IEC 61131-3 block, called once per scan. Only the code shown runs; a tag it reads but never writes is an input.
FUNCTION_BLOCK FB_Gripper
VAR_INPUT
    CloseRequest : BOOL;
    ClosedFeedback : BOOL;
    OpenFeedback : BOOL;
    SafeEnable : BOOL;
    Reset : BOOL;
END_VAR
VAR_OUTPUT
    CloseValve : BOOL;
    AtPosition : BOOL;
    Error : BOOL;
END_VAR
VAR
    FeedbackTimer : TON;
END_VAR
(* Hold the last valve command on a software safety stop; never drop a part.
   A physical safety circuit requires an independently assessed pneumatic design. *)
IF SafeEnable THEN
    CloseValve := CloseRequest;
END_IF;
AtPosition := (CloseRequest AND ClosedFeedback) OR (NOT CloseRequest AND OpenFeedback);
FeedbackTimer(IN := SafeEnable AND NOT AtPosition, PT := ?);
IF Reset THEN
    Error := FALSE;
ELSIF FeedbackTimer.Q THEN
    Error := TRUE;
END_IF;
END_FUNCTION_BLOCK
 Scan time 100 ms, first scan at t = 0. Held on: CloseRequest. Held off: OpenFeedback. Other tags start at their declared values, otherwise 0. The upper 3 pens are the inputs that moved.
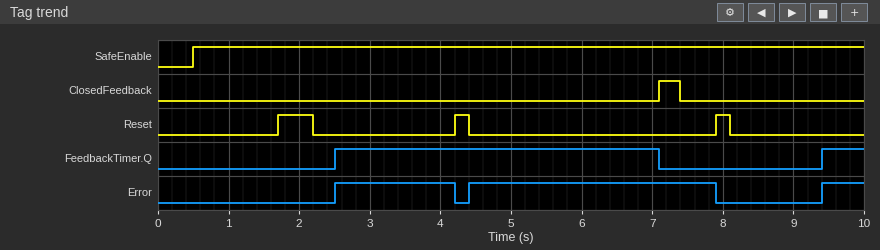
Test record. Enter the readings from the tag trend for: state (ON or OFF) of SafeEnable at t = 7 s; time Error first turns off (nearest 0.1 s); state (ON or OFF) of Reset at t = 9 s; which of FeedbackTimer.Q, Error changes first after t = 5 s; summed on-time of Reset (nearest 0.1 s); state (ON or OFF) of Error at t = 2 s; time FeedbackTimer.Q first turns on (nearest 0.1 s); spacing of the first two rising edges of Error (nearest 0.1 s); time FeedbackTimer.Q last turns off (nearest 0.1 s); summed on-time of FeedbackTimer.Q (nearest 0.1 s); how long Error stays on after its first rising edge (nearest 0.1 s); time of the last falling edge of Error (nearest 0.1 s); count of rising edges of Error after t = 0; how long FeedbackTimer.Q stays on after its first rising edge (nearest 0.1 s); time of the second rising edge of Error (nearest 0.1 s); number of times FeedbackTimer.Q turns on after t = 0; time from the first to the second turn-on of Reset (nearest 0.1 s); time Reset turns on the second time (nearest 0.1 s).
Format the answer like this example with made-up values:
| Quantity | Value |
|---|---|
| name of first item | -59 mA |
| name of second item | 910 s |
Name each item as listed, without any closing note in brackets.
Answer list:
| Quantity | Value |
|---|---|
| state (ON or OFF) of SafeEnable at t = 7 s | ON |
| time Error first turns off | 4.2 s |
| state (ON or OFF) of Reset at t = 9 s | OFF |
| which of FeedbackTimer.Q, Error changes first after t = 5 s | FeedbackTimer.Q |
| summed on-time of Reset | 0.9 s |
| state (ON or OFF) of Error at t = 2 s | OFF |
| time FeedbackTimer.Q first turns on | 2.5 s |
| spacing of the first two rising edges of Error | 1.9 s |
| time FeedbackTimer.Q last turns off | 7.1 s |
| summed on-time of FeedbackTimer.Q | 5.2 s |
| how long Error stays on after its first rising edge | 1.7 s |
| time of the last falling edge of Error | 7.9 s |
| count of rising edges of Error after t = 0 | 3 |
| how long FeedbackTimer.Q stays on after its first rising edge | 4.6 s |
| time of the second rising edge of Error | 4.4 s |
| number of times FeedbackTimer.Q turns on after t = 0 | 2 |
| time from the first to the second turn-on of Reset | 2.5 s |
| time Reset turns on the second time | 4.2 s |
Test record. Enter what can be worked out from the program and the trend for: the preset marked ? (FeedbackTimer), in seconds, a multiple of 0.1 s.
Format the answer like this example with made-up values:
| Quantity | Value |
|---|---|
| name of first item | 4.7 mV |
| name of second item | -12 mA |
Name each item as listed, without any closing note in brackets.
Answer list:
| Quantity | Value |
|---|---|
| the preset marked ? (FeedbackTimer), in seconds, a multiple of 0.1 s | 2.0 s |
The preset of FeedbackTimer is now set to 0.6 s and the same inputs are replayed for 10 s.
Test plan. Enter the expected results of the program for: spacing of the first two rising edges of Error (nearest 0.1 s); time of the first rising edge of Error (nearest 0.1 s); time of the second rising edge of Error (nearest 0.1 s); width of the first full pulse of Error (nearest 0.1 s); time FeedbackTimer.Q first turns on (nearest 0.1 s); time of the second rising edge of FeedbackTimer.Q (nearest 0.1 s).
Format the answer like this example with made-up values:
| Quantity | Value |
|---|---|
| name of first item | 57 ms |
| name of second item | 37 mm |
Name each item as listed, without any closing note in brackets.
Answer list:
| Quantity | Value |
|---|---|
| spacing of the first two rising edges of Error | 1.1 s |
| time of the first rising edge of Error | 1.1 s |
| time of the second rising edge of Error | 2.2 s |
| width of the first full pulse of Error | 0.6 s |
| time FeedbackTimer.Q first turns on | 1.1 s |
| time of the second rising edge of FeedbackTimer.Q | 8.0 s |
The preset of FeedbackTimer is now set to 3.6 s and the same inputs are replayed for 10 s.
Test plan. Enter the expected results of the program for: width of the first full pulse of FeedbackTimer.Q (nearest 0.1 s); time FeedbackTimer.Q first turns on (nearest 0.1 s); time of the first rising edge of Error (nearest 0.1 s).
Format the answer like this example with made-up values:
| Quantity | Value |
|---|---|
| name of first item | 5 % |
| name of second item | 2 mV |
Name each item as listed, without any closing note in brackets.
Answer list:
| Quantity | Value |
|---|---|
| width of the first full pulse of FeedbackTimer.Q | 3.0 s |
| time FeedbackTimer.Q first turns on | 4.1 s |
| time of the first rising edge of Error | 4.1 s |
